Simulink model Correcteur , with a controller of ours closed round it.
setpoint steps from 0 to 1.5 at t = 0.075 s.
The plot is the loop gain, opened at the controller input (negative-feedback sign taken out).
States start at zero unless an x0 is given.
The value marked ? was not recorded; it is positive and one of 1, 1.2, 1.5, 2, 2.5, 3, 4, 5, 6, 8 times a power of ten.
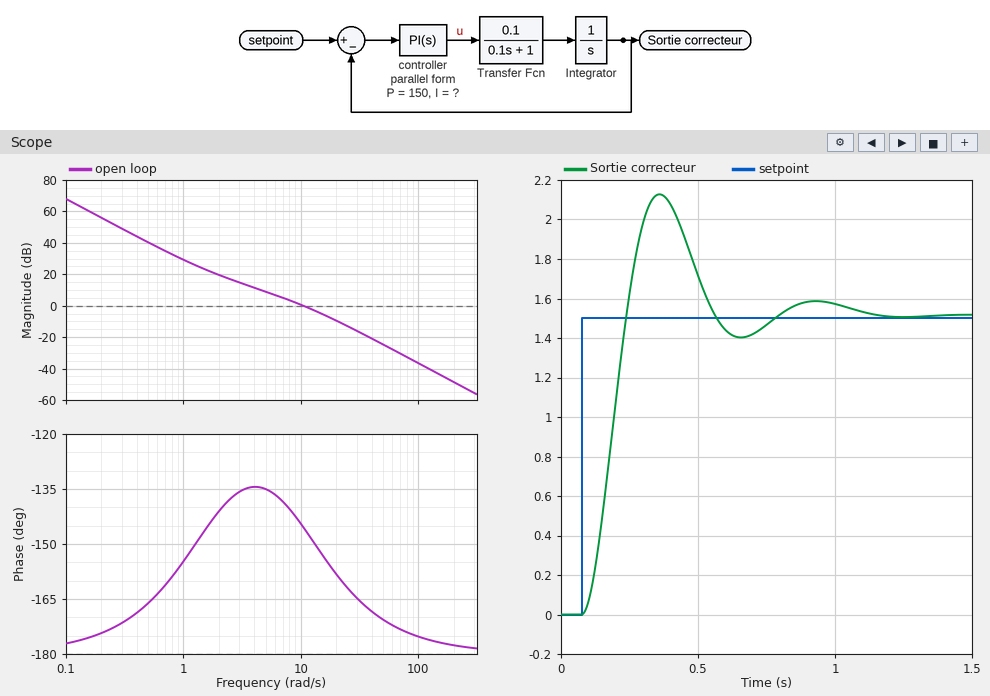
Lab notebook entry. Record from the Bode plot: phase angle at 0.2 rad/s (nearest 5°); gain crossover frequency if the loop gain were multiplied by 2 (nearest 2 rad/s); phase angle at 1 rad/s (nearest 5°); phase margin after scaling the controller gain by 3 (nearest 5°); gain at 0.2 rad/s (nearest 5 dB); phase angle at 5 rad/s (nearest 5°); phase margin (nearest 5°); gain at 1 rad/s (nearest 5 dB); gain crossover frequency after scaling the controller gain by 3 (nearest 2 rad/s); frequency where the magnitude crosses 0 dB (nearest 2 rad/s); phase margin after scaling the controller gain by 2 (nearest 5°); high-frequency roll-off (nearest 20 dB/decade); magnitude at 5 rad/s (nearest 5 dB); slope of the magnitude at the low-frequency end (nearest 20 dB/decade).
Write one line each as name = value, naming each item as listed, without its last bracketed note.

phase angle at 0.2 rad/s = -175°
gain crossover frequency if the loop gain were multiplied by 2 = 16 rad/s
phase angle at 1 rad/s = -155°
phase margin after scaling the controller gain by 3 = 20°
gain at 0.2 rad/s = 55 dB
phase angle at 5 rad/s = -135°
phase margin = 35°
gain at 1 rad/s = 30 dB
gain crossover frequency after scaling the controller gain by 3 = 20 rad/s
frequency where the magnitude crosses 0 dB = 10 rad/s
phase margin after scaling the controller gain by 2 = 25°
high-frequency roll-off = -40 dB/decade
magnitude at 5 rad/s = 10 dB
slope of the magnitude at the low-frequency end = -40 dB/decade
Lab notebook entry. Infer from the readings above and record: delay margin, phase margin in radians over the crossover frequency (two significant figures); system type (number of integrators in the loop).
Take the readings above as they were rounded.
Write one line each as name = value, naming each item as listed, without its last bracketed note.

delay margin, phase margin in radians over the crossover frequency = 0.061 s
system type = 2
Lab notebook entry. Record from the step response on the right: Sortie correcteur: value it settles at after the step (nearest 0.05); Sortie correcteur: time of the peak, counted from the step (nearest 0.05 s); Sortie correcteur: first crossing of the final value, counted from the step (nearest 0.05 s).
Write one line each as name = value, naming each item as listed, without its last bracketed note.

Sortie correcteur: value it settles at after the step = 1.50
Sortie correcteur: time of the peak, counted from the step = 0.30 s
Sortie correcteur: first crossing of the final value, counted from the step = 0.15 s
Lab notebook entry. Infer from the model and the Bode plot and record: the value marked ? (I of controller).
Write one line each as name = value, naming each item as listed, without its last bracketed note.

the value marked ? = 250
